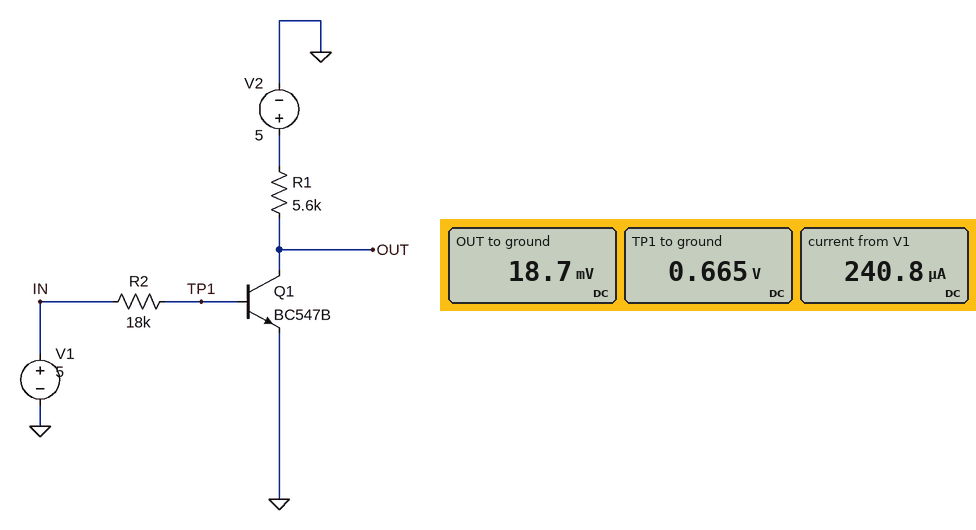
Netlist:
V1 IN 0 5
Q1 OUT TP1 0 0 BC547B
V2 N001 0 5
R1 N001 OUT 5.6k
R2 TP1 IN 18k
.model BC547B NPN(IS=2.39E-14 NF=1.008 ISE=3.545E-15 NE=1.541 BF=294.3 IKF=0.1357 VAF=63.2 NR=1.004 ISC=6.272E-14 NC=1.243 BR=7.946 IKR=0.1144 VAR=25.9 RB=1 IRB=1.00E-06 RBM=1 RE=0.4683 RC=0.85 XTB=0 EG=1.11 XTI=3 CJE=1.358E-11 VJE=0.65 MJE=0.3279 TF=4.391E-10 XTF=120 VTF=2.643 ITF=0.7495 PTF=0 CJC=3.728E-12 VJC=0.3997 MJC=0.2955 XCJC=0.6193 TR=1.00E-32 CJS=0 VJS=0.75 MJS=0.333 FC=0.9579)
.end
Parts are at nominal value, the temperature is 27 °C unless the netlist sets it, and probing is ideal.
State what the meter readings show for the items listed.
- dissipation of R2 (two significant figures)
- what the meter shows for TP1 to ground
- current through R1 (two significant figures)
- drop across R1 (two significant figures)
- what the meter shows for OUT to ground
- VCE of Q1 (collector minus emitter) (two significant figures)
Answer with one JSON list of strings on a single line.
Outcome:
["1.0 mW", "0.665 V", "890 µA", "5.0 V", "18.7 mV", "19 mV"]
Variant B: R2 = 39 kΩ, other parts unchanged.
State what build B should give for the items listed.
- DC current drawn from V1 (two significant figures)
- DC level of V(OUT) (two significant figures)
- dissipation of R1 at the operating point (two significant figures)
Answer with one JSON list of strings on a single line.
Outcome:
["110 µA", "28 mV", "4.4 mW"]
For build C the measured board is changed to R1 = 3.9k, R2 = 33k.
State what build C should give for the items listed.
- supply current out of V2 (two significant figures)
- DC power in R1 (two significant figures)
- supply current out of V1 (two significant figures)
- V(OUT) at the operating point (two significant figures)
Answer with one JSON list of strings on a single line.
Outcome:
["1.3 mA", "6.3 mW", "130 µA", "31 mV"]
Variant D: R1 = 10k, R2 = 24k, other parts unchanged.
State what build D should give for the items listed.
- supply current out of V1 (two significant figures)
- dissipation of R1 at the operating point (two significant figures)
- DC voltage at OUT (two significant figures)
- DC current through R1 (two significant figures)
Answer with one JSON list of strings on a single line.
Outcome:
["180 µA", "2.5 mW", "16 mV", "500 µA"]
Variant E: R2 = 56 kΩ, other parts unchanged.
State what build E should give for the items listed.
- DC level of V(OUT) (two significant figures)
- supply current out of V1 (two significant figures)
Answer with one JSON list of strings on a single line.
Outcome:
["33 mV", "78 µA"]
